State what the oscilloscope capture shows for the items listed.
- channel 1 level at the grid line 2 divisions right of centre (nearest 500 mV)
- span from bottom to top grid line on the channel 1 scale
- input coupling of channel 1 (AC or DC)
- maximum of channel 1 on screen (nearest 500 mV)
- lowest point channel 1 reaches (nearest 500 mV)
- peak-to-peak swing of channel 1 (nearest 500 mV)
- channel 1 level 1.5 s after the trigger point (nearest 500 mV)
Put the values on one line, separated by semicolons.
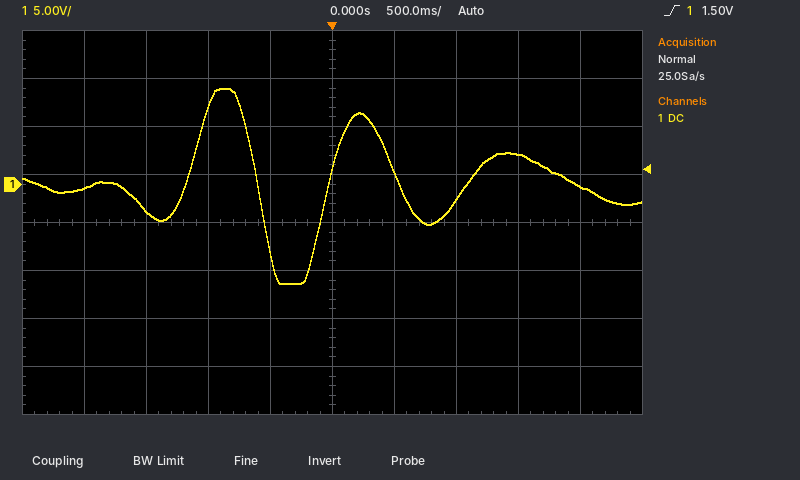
-1.5 V; 40 V; DC; 10.0 V; -10.5 V; 20.5 V; 3.0 V
